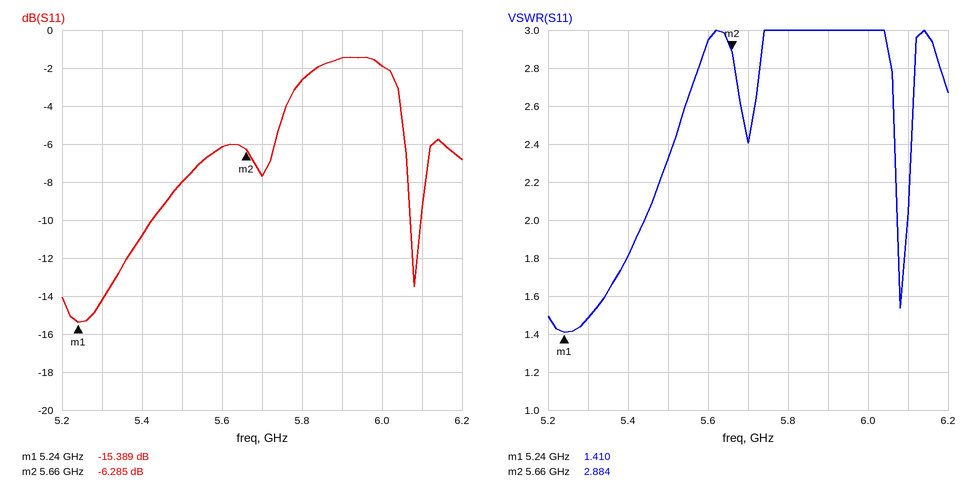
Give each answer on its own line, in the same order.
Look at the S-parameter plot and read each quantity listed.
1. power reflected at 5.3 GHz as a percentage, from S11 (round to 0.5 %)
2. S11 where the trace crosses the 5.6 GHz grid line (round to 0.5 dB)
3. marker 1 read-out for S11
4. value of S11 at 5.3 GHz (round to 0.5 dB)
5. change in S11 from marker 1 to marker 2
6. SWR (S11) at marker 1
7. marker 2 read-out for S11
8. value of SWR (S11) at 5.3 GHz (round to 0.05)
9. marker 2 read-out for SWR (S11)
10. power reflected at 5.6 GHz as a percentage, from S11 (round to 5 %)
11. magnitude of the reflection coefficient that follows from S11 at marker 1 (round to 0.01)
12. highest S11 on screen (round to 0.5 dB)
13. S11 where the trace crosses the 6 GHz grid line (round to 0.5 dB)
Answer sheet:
4.0 %
-6.0 dB
-15.389 dB
-14.0 dB
9.104 dB
1.410
-6.285 dB
1.50
2.884
25 %
0.17
-1.5 dB
-2.0 dB
